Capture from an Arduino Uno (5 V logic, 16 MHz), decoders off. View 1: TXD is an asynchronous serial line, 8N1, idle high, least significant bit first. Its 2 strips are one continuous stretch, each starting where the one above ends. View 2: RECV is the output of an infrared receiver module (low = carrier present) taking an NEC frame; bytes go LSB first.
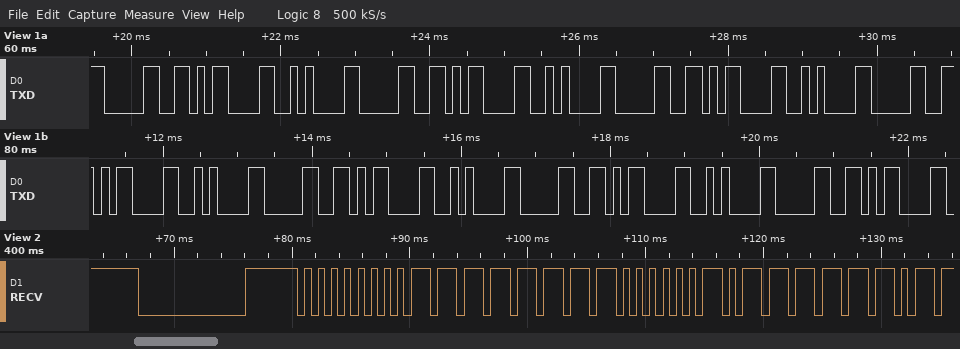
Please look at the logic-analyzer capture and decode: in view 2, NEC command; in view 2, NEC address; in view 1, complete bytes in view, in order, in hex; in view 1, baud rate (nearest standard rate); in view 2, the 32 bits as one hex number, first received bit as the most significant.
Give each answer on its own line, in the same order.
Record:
0x40
0x00
0x30 0x0D 0x0A 0x30 0x0D 0x0A 0x30 0x0D 0x0A 0x30 0x0D 0x0A 0x30 0x0D 0x0A 0x30 0x0D 0x0A 0x30 0x0D
9600 baud
0x00FF02FD
